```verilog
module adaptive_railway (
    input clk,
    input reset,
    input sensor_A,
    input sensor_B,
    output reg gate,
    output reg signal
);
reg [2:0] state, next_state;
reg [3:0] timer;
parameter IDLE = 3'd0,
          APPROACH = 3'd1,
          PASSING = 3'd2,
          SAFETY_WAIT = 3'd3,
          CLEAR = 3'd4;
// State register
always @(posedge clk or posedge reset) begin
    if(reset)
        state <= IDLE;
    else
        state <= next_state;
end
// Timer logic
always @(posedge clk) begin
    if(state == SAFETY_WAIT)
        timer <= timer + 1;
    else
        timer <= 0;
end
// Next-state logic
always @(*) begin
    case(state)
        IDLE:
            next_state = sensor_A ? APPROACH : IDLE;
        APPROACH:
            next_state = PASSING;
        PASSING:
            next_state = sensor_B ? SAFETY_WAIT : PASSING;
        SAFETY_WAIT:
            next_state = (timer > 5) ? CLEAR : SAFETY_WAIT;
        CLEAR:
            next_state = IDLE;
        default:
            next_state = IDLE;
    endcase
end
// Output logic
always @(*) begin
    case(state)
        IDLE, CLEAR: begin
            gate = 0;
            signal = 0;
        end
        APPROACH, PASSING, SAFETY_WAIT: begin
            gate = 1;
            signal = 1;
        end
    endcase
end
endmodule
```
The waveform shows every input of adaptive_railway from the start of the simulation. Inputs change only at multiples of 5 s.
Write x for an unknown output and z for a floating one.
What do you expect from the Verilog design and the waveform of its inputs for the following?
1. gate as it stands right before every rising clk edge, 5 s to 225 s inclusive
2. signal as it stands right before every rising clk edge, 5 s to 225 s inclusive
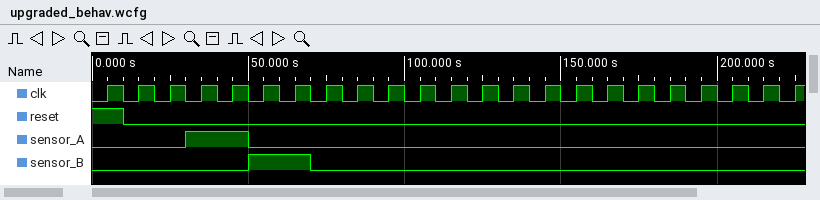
0 0 0 0 1 1 1 1 1 1 1 1 1 0 0 0 0 0 0 0 0 0 0
0 0 0 0 1 1 1 1 1 1 1 1 1 0 0 0 0 0 0 0 0 0 0
